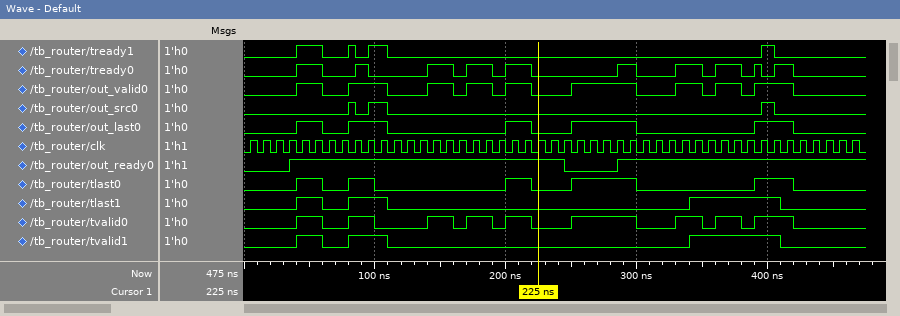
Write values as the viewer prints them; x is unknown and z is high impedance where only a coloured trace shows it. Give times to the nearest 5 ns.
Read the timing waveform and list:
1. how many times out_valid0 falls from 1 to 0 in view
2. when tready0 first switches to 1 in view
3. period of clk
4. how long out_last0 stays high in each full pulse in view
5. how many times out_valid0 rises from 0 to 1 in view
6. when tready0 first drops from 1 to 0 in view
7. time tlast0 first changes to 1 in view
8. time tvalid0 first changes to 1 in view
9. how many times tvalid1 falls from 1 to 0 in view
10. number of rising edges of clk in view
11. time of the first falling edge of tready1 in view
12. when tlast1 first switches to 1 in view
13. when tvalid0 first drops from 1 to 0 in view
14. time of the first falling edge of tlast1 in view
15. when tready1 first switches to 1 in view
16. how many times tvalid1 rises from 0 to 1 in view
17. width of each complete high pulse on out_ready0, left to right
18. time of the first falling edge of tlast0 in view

9
40 ns
10 ns
20 ns, 30 ns, 20 ns, 50 ns, 30 ns
9
60 ns
40 ns
40 ns
3
47
60 ns
40 ns
60 ns
60 ns
40 ns
3
210 ns
60 ns
